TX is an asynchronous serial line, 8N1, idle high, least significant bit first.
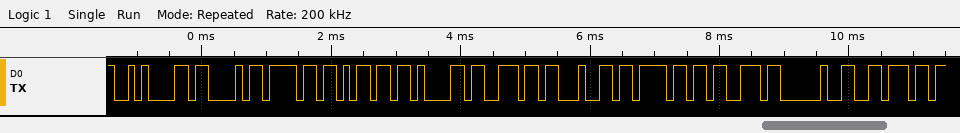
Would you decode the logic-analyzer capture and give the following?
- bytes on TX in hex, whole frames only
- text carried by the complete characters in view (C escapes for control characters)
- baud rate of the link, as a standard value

0x0A 0x43 0x6F 0x6D 0x61 0x6E 0x64 0x6F 0x73 0x20 0x76
"\nComandos v"
9600 baud
